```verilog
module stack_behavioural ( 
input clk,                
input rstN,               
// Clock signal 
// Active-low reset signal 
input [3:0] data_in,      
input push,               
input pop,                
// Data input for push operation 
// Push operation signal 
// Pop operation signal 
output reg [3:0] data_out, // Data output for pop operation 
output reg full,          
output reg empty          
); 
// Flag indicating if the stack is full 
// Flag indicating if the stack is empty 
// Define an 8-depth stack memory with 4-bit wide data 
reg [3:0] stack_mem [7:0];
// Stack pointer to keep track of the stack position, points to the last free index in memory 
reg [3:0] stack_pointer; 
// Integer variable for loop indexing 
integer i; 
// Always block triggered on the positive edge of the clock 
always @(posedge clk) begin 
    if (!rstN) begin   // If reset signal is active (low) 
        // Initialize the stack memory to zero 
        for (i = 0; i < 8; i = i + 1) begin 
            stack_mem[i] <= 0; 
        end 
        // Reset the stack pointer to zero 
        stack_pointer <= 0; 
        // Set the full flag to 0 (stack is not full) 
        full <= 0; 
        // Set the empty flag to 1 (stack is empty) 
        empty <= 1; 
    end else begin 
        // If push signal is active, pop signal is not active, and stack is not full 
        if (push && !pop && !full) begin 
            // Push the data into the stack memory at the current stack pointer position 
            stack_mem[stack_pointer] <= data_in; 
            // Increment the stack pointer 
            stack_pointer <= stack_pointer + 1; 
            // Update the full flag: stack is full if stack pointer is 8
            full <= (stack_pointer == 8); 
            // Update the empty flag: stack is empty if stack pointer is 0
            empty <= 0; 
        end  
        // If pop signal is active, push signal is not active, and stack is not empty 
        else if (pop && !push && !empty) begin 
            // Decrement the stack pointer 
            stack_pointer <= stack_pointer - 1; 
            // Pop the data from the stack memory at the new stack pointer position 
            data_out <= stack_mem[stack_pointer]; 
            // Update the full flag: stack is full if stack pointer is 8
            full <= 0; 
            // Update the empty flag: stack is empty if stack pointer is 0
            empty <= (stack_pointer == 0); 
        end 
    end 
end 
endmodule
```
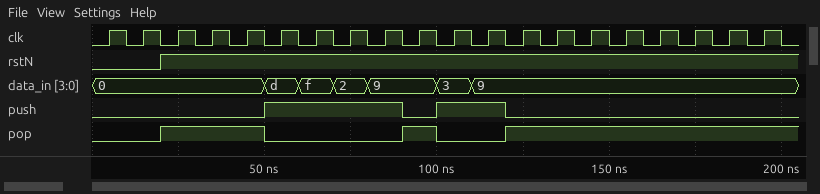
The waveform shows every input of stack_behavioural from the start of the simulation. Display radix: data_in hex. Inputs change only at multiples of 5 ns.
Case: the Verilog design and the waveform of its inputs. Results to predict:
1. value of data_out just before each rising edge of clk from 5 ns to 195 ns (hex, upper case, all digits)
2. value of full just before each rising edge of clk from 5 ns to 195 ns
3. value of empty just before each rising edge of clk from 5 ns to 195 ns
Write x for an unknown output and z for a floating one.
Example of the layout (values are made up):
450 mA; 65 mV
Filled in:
x, x, x, x, x, x, x, x, x, x, 0, 0, 0, 0, 9, 3, 2, F, D, D; x 0 0 0 0 0 0 0 0 0 0 0 0 0 0 0 0 0 0 0; x 1 1 1 1 1 0 0 0 0 0 0 0 0 0 0 0 0 1 1
